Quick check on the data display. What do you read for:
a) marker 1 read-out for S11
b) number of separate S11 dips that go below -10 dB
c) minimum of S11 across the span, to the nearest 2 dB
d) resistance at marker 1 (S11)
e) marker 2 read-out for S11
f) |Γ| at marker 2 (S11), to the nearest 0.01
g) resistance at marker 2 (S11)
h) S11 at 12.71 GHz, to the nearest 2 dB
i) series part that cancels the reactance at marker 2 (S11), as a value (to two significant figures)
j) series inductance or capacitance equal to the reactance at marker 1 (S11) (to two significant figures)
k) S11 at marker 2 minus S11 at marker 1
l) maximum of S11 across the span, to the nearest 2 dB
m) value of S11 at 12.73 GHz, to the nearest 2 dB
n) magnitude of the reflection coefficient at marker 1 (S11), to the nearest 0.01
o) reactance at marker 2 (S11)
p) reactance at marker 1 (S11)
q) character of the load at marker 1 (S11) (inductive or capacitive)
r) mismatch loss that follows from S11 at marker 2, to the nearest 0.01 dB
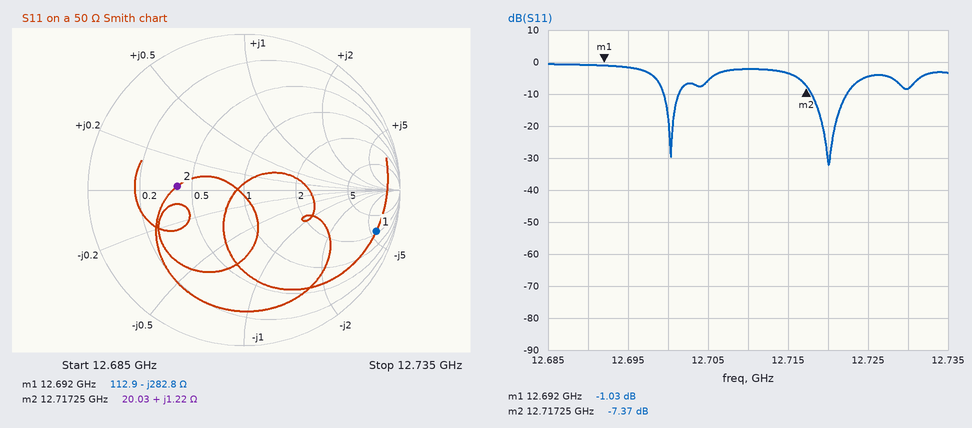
-1.03 dB
2
-32 dB
112.9 Ω
-7.37 dB
0.43
20.03 Ω
-2 dB
10 pF
44 fF
-6.34 dB
0 dB
-8 dB
0.89
+1.22 Ω
-282.8 Ω
capacitive
0.88 dB
